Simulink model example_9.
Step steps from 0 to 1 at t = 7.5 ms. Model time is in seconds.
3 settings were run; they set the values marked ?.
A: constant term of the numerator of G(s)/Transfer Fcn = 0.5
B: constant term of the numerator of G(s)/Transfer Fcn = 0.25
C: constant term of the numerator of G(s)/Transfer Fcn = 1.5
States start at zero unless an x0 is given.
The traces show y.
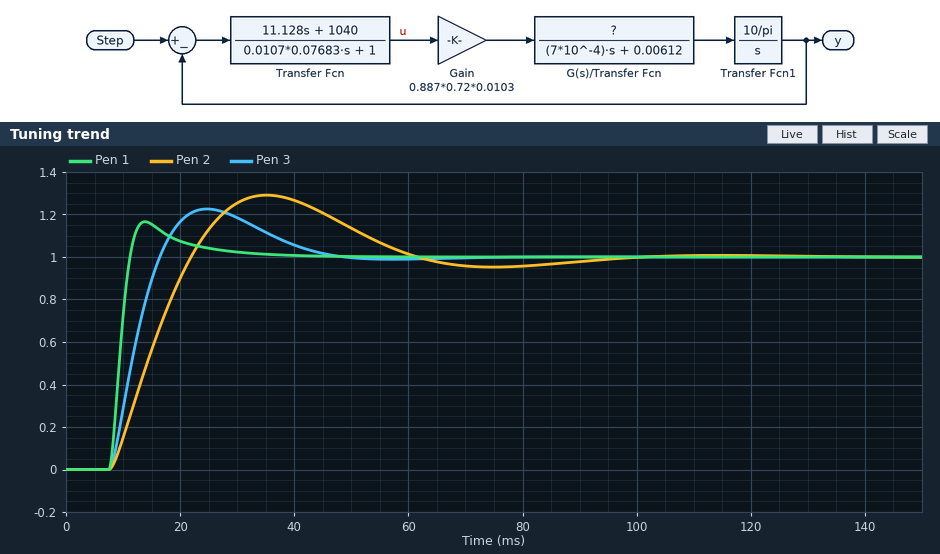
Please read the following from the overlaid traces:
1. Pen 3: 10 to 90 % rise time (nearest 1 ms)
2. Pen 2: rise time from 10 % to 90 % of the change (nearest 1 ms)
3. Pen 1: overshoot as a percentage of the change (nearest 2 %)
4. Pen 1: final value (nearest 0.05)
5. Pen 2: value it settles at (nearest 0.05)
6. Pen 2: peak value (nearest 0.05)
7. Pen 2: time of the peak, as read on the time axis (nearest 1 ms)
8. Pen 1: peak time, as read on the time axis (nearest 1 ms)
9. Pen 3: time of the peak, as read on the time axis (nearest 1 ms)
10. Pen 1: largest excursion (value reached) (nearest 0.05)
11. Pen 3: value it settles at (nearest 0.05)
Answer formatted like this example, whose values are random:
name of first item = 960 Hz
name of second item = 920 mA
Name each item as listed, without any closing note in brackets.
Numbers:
Pen 3: 10 to 90 % rise time = 6 ms
Pen 2: rise time from 10 % to 90 % of the change = 11 ms
Pen 1: overshoot as a percentage of the change = 16 %
Pen 1: final value = 1.00
Pen 2: value it settles at = 1.00
Pen 2: peak value = 1.30
Pen 2: time of the peak, as read on the time axis = 35 ms
Pen 1: peak time, as read on the time axis = 14 ms
Pen 3: time of the peak, as read on the time axis = 25 ms
Pen 1: largest excursion (value reached) = 1.15
Pen 3: value it settles at = 1.00
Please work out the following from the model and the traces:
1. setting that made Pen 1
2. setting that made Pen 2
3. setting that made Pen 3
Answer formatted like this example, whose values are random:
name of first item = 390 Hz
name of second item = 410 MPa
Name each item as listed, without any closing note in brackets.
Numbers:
setting that made Pen 1 = C
setting that made Pen 2 = B
setting that made Pen 3 = A
